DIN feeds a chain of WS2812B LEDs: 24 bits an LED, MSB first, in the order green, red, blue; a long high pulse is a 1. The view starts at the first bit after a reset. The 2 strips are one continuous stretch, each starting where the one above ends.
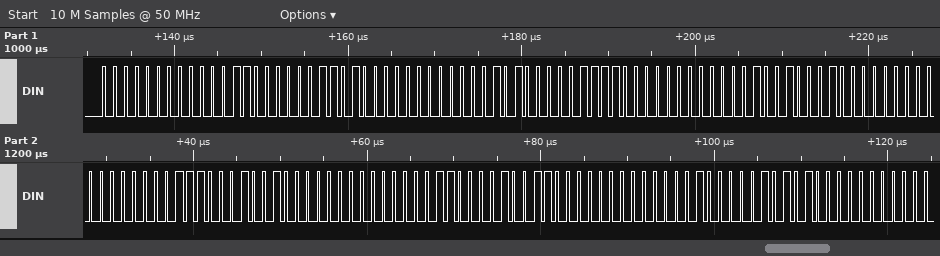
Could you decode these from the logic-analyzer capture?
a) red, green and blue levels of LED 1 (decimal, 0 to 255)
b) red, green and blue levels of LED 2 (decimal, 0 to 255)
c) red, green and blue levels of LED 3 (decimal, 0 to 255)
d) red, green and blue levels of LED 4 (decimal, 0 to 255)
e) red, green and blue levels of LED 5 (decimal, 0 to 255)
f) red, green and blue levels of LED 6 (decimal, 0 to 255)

12, 0, 13
10, 0, 15
9, 0, 16
7, 0, 18
6, 0, 19
4, 0, 21
